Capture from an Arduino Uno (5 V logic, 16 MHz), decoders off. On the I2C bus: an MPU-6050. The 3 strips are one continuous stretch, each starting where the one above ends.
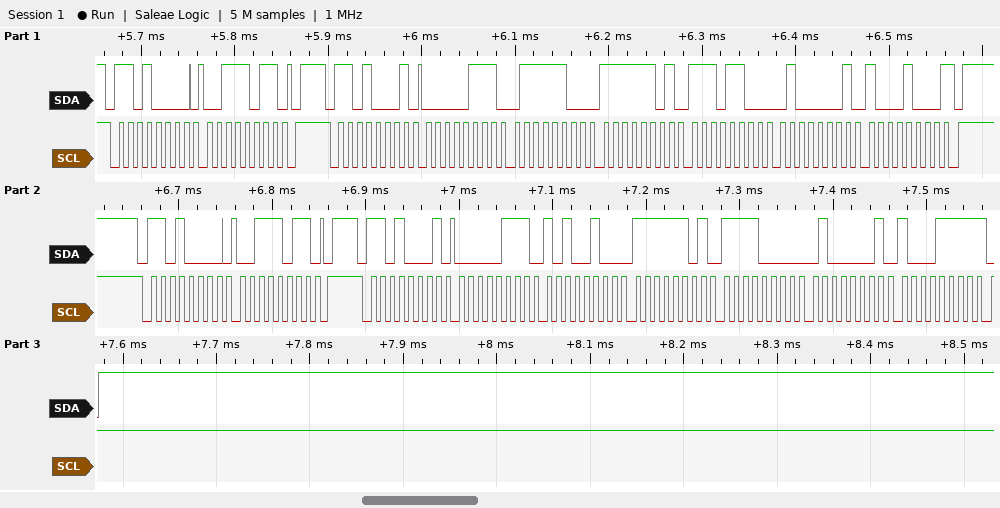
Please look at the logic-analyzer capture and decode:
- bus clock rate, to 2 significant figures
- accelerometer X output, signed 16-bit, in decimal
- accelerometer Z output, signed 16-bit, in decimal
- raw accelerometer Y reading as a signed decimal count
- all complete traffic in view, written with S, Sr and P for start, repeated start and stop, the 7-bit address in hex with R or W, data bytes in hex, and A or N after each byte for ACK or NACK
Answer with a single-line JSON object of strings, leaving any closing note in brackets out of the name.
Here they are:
{"bus clock rate, to 2 significant figures": "100 kHz", "accelerometer X output, signed 16-bit, in decimal": "1916", "accelerometer Z output, signed 16-bit, in decimal": "16776", "raw accelerometer Y reading as a signed decimal count": "-532", "all complete traffic in view, written with S, Sr and P for start, repeated start and stop, the 7-bit address in hex with R or W, data bytes in hex, and A or N after each byte for ACK or NACK": "S 68W A 3B A P S 68R A 07 A 7C A FD A EC A 41 A 88 N P S 68W A 3B A P S 68R A 07 A A4 A FD A F0 A 41 A 8F N P"}
